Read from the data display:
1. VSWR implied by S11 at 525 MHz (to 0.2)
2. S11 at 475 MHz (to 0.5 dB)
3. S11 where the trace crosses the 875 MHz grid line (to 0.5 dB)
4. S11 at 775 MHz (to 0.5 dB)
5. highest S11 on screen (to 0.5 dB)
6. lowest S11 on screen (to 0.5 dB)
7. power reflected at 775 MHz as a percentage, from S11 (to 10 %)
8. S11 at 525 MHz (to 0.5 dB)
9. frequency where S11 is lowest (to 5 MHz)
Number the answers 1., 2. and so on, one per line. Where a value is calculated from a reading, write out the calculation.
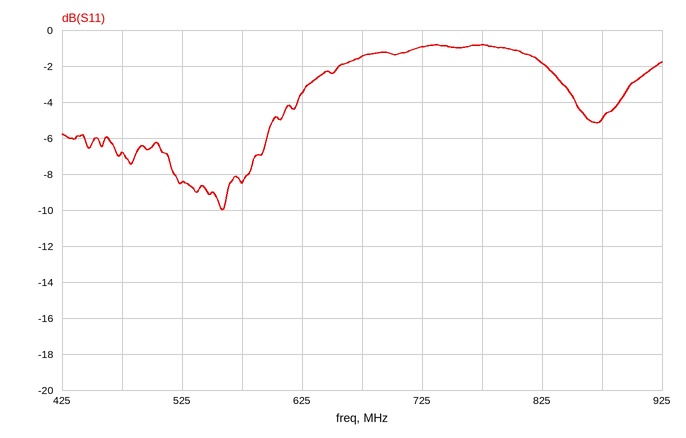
1. |Γ| = 10^(-8.5/20) = 0.3758; VSWR = (1 + 0.3758)/(1 − 0.3758) ≈ 2.2
2. -7.0 dB
3. -5.0 dB
4. -1.0 dB
5. -1.0 dB
6. -10.0 dB
7. 10^(-1/10) ≈ 79.4 %, so 80 % to the nearest 10 %
8. -8.5 dB
9. 560 MHz
